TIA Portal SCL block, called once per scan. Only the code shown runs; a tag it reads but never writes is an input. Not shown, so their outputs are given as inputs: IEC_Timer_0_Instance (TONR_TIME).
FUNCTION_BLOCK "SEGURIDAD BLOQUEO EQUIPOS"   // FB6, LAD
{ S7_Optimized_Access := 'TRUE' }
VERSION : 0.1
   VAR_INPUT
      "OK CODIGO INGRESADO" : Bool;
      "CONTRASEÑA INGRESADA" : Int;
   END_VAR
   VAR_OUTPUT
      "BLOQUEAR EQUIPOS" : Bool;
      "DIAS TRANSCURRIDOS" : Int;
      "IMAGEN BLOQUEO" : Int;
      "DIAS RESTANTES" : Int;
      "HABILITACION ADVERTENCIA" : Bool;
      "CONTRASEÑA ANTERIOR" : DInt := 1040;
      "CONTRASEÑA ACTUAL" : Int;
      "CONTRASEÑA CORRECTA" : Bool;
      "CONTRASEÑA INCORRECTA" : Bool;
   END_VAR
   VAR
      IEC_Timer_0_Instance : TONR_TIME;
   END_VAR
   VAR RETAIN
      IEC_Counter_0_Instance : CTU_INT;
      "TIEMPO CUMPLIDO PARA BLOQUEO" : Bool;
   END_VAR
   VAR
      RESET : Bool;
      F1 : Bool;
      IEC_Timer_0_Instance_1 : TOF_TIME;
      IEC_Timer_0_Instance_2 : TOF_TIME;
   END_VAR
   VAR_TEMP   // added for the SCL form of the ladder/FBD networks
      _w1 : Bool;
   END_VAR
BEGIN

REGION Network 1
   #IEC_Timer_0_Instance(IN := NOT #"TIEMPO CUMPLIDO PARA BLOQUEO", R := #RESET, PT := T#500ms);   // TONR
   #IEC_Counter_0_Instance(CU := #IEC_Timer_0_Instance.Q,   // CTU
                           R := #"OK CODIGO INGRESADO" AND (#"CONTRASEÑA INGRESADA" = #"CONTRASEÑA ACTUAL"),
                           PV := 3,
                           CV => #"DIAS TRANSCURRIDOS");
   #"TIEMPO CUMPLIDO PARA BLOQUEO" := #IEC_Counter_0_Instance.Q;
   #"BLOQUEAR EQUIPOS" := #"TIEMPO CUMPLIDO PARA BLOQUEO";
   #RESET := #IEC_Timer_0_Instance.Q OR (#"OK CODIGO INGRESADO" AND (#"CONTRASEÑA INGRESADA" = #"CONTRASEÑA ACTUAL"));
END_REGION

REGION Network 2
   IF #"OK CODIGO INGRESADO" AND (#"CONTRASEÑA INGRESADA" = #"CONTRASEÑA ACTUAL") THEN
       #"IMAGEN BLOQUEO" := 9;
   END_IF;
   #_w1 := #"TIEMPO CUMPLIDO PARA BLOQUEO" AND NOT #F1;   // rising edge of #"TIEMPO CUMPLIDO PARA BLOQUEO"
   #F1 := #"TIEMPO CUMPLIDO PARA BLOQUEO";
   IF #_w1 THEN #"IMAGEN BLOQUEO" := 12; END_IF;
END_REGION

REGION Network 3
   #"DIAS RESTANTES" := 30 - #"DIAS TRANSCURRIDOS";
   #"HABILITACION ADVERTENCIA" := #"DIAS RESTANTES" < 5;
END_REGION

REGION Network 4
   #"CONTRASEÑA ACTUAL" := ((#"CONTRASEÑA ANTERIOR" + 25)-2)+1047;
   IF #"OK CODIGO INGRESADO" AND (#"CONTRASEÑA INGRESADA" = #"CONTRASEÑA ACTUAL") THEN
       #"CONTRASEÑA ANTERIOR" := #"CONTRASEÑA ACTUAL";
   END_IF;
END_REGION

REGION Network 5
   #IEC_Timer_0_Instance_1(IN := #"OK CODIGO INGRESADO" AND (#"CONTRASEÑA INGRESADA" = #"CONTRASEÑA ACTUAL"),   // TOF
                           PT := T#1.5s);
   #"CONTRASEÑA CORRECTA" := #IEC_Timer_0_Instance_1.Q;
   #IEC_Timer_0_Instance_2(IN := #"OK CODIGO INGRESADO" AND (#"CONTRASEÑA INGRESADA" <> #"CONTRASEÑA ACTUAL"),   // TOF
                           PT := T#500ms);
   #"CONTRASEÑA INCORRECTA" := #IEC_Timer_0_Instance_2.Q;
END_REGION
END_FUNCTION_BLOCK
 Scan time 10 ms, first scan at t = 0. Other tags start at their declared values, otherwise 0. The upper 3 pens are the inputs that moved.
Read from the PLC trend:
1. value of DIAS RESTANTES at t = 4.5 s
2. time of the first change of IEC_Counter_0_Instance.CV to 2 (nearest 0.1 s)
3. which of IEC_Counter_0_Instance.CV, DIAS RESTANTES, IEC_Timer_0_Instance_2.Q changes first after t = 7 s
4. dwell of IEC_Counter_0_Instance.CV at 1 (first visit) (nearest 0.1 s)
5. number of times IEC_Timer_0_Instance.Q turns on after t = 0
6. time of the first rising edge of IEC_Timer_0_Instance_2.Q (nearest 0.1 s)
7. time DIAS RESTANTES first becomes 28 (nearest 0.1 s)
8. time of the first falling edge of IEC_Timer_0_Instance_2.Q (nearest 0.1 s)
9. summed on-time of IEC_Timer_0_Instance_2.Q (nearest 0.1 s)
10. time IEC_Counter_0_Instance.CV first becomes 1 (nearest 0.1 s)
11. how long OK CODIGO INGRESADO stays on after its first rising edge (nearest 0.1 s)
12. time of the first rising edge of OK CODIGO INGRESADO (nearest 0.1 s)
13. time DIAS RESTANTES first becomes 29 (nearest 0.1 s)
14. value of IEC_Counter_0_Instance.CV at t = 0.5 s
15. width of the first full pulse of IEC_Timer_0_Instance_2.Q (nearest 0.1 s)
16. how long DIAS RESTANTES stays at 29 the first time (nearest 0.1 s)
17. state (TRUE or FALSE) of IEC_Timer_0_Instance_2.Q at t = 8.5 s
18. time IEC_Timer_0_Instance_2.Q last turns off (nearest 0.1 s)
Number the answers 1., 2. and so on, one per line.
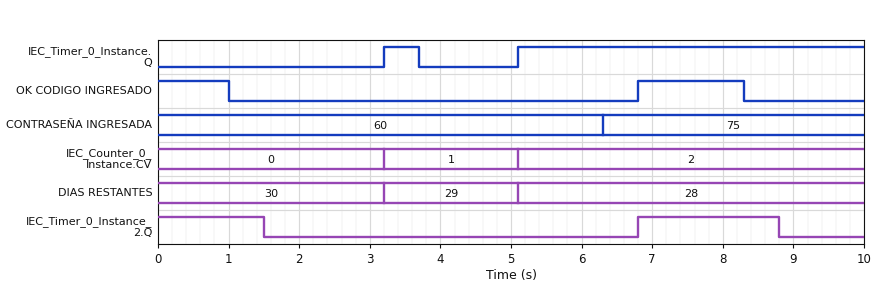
1. 29
2. 5.1 s
3. IEC_Timer_0_Instance_2.Q
4. 1.9 s
5. 2
6. 6.8 s
7. 5.1 s
8. 1.5 s
9. 3.5 s
10. 3.2 s
11. 1.5 s
12. 6.8 s
13. 3.2 s
14. 0
15. 2.0 s
16. 1.9 s
17. TRUE
18. 8.8 s
